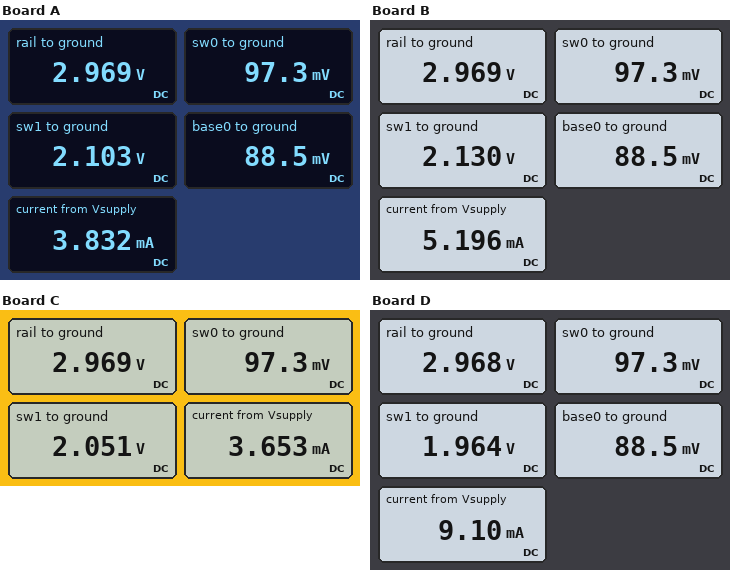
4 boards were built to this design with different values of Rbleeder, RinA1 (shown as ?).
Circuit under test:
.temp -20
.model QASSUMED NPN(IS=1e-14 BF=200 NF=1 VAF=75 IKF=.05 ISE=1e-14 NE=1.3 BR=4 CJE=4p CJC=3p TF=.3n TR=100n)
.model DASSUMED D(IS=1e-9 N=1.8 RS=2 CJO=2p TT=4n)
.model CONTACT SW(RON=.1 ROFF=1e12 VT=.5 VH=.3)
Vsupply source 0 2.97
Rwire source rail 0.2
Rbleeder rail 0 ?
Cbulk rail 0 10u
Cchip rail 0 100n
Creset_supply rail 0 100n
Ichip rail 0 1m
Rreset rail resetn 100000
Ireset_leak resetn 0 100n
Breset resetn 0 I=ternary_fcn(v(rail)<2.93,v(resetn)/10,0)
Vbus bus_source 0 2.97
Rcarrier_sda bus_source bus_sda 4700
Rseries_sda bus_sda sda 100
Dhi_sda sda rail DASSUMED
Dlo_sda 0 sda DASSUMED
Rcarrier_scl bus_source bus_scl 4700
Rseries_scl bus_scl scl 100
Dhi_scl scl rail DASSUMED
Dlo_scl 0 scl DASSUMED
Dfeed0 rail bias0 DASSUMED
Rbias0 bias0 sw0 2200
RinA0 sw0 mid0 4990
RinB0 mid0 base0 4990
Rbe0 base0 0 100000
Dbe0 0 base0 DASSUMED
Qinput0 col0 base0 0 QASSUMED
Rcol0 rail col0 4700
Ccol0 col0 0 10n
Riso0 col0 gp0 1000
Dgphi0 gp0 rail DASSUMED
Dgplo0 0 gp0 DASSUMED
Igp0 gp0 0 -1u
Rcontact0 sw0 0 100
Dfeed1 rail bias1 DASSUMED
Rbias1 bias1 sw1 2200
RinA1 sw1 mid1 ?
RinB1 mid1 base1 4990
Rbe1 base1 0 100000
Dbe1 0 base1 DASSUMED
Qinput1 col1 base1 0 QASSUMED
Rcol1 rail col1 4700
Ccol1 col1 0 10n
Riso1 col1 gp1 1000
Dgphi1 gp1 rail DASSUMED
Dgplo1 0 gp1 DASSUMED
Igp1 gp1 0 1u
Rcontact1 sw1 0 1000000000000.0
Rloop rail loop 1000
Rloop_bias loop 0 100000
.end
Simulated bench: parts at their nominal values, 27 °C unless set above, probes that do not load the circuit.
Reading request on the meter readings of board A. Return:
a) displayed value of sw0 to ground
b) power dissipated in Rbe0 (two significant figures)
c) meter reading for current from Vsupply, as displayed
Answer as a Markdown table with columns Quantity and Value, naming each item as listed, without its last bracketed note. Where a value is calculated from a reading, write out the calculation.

| Quantity | Value |
|---|---|
| displayed value of sw0 to ground | 97.3 mV |
| power dissipated in Rbe0 | (88.5 mV)^2 / 100 kΩ = 78 nW |
| meter reading for current from Vsupply, as displayed | 3.832 mA |
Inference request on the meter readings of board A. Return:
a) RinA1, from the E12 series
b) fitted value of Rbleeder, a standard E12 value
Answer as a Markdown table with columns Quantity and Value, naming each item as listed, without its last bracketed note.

| Quantity | Value |
|---|---|
| RinA1, from the E12 series | 8.2 kΩ |
| fitted value of Rbleeder, a standard E12 value | 2.7 kΩ |
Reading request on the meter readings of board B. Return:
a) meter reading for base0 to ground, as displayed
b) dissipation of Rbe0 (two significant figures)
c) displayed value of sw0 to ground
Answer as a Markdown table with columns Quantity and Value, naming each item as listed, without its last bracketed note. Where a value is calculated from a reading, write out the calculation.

| Quantity | Value |
|---|---|
| meter reading for base0 to ground, as displayed | 88.5 mV |
| dissipation of Rbe0 | (88.5 mV)^2 / 100 kΩ = 78 nW |
| displayed value of sw0 to ground | 97.3 mV |
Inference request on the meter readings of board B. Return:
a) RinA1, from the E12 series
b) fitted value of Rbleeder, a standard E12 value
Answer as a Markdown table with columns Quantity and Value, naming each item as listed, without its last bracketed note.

| Quantity | Value |
|---|---|
| RinA1, from the E12 series | 10 kΩ |
| fitted value of Rbleeder, a standard E12 value | 1.2 kΩ |
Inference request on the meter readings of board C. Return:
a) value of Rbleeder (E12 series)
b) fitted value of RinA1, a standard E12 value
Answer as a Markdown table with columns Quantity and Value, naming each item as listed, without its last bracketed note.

| Quantity | Value |
|---|---|
| value of Rbleeder | 3.3 kΩ |
| fitted value of RinA1, a standard E12 value | 5.6 kΩ |
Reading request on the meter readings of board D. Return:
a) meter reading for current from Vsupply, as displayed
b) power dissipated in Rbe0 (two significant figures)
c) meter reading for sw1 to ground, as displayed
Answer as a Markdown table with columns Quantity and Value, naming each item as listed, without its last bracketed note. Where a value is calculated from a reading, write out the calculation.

| Quantity | Value |
|---|---|
| meter reading for current from Vsupply, as displayed | 9.10 mA |
| power dissipated in Rbe0 | (88.5 mV)^2 / 100 kΩ = 78 nW |
| meter reading for sw1 to ground, as displayed | 1.964 V |
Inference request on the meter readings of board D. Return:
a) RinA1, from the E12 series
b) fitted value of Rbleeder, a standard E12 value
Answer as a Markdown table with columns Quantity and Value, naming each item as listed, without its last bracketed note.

| Quantity | Value |
|---|---|
| RinA1, from the E12 series | 2.7 kΩ |
| fitted value of Rbleeder, a standard E12 value | 470 Ω |
